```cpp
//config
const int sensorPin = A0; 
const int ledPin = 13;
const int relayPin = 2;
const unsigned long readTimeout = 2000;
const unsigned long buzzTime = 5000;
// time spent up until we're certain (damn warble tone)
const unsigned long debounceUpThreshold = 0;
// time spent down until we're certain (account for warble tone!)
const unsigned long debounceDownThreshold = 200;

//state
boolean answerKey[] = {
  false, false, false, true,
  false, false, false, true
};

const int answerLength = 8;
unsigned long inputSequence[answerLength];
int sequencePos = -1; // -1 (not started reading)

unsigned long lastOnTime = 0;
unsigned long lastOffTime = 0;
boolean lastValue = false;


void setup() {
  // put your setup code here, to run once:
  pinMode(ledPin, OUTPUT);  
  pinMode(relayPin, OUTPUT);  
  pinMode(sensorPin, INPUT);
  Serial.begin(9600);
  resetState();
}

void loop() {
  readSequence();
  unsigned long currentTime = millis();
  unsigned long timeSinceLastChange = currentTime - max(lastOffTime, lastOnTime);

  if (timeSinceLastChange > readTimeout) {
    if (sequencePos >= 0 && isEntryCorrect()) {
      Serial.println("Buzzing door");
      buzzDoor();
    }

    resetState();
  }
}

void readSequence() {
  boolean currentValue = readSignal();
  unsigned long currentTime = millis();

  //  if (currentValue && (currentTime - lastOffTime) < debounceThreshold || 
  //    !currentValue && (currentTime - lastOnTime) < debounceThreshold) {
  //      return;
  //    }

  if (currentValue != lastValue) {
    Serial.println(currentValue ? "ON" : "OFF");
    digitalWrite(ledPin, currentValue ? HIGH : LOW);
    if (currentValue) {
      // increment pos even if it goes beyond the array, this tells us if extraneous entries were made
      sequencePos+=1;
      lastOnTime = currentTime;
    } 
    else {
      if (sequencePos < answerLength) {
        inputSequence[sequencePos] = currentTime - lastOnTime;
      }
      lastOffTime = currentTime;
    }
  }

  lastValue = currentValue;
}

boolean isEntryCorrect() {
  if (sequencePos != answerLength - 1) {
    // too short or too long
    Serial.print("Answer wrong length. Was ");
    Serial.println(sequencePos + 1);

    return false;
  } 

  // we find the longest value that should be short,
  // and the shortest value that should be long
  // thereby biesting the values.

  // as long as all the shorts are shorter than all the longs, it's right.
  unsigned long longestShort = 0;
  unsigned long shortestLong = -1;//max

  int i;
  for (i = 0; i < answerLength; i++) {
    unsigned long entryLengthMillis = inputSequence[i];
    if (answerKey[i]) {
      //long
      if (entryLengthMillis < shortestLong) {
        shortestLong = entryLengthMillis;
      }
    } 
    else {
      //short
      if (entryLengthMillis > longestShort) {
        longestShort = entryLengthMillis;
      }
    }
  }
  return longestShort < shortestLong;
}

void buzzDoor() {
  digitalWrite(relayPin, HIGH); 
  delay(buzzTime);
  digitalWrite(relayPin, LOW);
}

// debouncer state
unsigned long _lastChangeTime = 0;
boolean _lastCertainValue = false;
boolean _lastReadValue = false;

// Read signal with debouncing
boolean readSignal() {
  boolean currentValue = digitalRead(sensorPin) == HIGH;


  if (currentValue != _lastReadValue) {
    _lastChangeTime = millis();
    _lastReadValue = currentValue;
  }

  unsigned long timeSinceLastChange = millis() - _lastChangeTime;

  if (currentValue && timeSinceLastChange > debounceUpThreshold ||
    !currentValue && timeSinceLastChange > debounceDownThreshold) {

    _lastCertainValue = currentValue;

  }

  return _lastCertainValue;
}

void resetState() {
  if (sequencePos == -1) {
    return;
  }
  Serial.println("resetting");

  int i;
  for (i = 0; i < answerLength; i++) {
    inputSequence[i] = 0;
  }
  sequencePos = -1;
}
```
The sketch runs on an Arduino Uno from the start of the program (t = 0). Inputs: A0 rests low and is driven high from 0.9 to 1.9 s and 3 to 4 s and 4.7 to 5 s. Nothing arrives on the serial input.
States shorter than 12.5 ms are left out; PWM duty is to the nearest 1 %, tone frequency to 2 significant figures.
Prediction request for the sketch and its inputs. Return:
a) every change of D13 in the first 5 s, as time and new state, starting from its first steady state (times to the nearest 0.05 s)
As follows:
0 s low; 0.9 s high; 2.1 s low; 3 s high; 4.2 s low; 4.7 s high
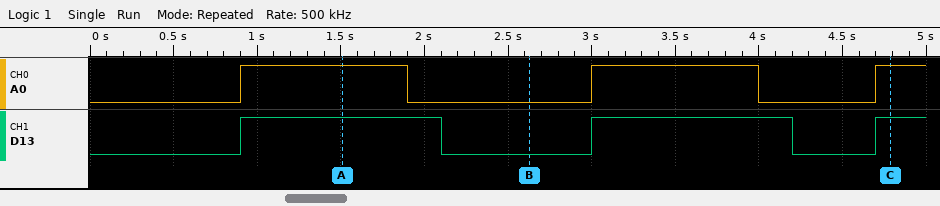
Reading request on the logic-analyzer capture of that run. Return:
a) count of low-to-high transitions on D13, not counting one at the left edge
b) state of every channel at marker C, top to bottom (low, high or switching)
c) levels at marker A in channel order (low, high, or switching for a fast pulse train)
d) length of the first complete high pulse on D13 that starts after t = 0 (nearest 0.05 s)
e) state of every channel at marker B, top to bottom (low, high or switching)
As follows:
3
A0 high, D13 high
A0 high, D13 high
1.20 s
A0 low, D13 low
